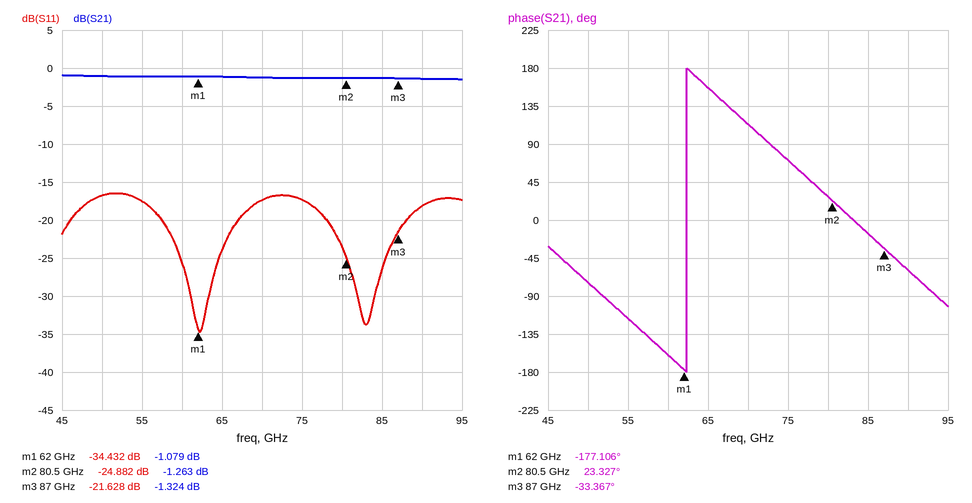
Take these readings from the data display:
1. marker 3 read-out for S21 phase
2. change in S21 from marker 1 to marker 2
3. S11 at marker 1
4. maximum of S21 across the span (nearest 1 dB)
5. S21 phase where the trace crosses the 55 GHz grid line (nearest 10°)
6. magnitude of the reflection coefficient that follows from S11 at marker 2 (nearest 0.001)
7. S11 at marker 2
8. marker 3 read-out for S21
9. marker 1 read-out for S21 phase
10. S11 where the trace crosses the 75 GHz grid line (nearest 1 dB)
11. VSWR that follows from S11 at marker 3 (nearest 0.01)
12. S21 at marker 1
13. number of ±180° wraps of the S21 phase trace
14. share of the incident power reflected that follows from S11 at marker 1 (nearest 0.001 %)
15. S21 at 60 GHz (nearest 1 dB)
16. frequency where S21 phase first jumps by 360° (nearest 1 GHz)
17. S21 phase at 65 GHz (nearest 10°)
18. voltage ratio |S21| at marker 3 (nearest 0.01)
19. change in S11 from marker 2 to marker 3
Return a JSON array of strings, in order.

["-33.367°", "-0.184 dB", "-34.432 dB", "-1 dB", "-120°", "0.057", "-24.882 dB", "-1.324 dB", "-177.106°", "-17 dB", "1.18", "-1.079 dB", "1", "0.036 %", "-1 dB", "62 GHz", "160°", "0.86", "3.254 dB"]
